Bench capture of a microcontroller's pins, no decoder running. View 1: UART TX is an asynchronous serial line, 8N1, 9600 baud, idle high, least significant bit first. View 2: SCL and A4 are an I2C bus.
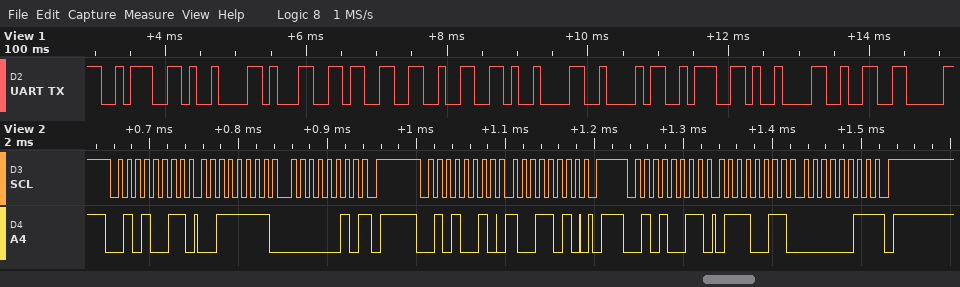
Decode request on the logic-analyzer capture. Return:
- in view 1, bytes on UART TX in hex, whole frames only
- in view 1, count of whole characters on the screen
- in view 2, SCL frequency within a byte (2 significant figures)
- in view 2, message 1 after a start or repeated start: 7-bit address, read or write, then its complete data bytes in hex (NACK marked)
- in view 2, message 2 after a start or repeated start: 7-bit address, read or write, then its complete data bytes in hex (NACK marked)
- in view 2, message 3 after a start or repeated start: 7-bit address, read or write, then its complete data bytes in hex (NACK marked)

3A 09 31 33 32 09 42 3A 09 32
10
100 kHz
0x29 read: 3F 02 NACK
0x29 write: 9A
0x29 read: 73 03 NACK
